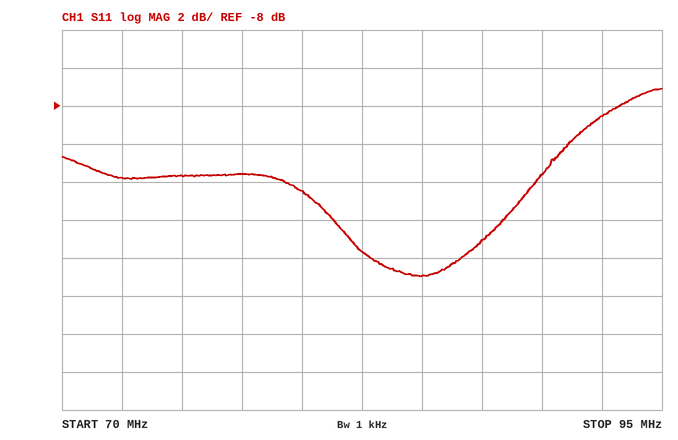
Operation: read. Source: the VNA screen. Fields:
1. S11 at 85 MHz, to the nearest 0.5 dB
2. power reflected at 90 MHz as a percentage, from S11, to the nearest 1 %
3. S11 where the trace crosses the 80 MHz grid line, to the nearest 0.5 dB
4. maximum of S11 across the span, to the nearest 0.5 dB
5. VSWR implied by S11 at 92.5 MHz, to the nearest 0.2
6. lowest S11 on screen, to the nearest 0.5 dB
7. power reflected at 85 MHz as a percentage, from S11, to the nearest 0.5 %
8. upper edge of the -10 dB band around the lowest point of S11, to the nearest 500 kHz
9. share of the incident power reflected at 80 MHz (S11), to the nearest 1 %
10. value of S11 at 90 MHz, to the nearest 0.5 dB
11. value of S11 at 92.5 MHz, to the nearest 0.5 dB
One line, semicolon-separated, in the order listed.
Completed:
-17.0 dB; 7 %; -12.5 dB; -7.0 dB; 2.2; -17.0 dB; 2.0 %; 91.0 MHz; 6 %; -11.5 dB; -8.5 dB
